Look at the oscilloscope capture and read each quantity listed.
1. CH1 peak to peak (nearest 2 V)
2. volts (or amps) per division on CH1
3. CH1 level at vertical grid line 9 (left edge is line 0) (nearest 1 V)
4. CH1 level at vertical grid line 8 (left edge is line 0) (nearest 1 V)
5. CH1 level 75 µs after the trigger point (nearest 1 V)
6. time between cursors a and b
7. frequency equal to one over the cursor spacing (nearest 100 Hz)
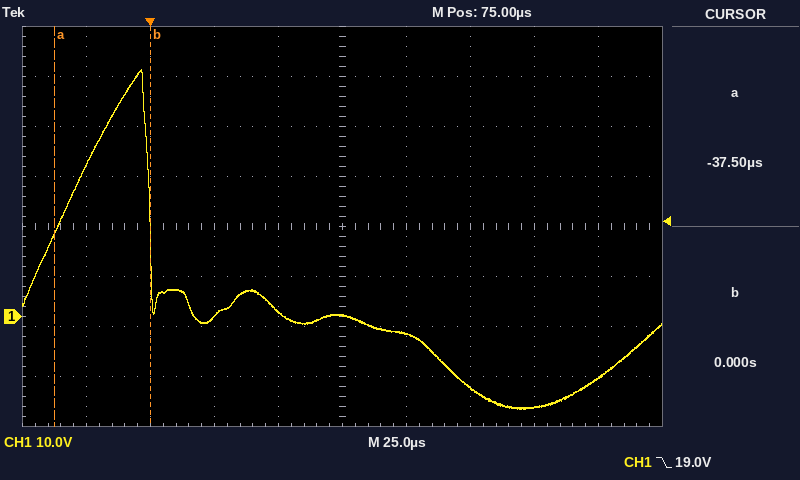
68 V
10 V
-12 V
-18 V
0 V
37.5 µs
26.7 kHz
